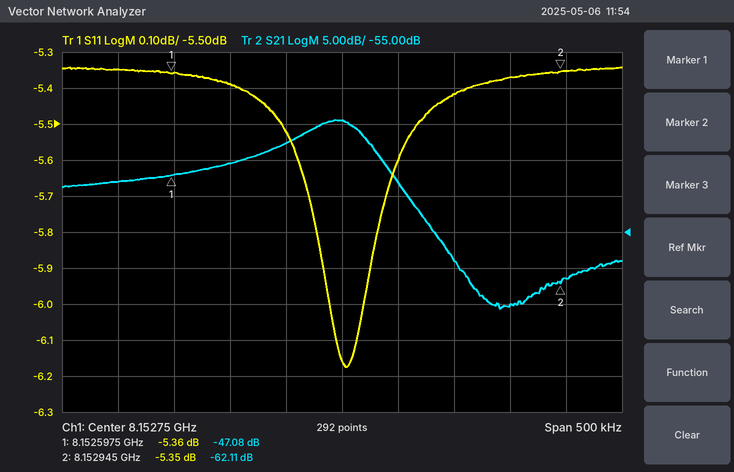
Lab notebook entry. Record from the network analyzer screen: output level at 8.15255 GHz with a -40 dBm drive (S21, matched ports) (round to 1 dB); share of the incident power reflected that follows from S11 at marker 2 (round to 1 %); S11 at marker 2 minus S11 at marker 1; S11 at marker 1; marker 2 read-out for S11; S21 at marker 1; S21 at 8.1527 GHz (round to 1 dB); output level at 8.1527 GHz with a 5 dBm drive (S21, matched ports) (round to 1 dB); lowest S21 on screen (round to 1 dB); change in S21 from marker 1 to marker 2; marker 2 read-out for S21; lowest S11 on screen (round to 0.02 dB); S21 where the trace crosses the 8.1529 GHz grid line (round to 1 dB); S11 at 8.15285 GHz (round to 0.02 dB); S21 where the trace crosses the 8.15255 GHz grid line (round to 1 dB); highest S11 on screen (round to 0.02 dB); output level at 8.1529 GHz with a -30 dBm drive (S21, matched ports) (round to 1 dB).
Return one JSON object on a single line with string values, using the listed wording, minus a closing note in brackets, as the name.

{"output level at 8.15255 GHz with a -40 dBm drive (S21, matched ports)": "-88 dBm", "share of the incident power reflected that follows from S11 at marker 2": "29 %", "S11 at marker 2 minus S11 at marker 1": "0.01 dB", "S11 at marker 1": "-5.36 dB", "marker 2 read-out for S11": "-5.35 dB", "S21 at marker 1": "-47.08 dB", "S21 at 8.1527 GHz": "-43 dB", "output level at 8.1527 GHz with a 5 dBm drive (S21, matched ports)": "-38 dBm", "lowest S21 on screen": "-66 dB", "change in S21 from marker 1 to marker 2": "-15.03 dB", "marker 2 read-out for S21": "-62.11 dB", "lowest S11 on screen": "-6.18 dB", "S21 where the trace crosses the 8.1529 GHz grid line": "-65 dB", "S11 at 8.15285 GHz": "-5.42 dB", "S21 where the trace crosses the 8.15255 GHz grid line": "-48 dB", "highest S11 on screen": "-5.34 dB", "output level at 8.1529 GHz with a -30 dBm drive (S21, matched ports)": "-95 dBm"}
